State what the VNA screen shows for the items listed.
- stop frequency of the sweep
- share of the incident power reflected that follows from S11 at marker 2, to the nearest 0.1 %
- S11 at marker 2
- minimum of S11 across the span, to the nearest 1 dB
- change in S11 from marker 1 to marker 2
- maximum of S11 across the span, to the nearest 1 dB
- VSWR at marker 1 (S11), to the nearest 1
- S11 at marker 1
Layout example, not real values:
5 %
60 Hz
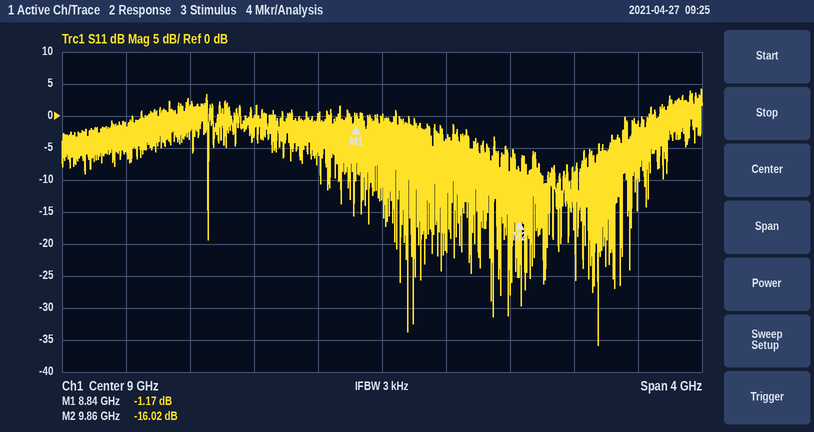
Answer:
11 GHz
2.5 %
-16.02 dB
-36 dB
-14.85 dB
4 dB
15
-1.17 dB
